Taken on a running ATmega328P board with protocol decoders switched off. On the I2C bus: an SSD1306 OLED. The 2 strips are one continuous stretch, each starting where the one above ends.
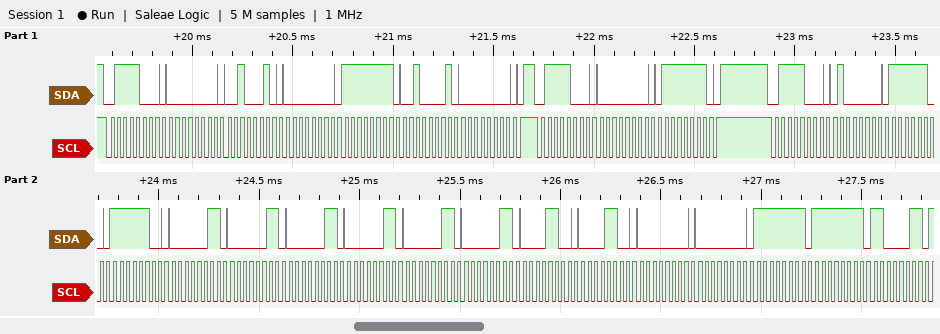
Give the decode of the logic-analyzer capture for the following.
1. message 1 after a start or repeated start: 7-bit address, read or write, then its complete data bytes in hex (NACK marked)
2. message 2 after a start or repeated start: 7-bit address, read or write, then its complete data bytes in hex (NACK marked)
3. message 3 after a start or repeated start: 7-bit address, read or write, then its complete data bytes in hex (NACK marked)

0x3C write: 00 22 00 FF 21 00
0x3C write: 00 7F
0x3C write: 40 FC FC 03 03 03 03 03 03 0C 0C 00 00 FF FF C3
